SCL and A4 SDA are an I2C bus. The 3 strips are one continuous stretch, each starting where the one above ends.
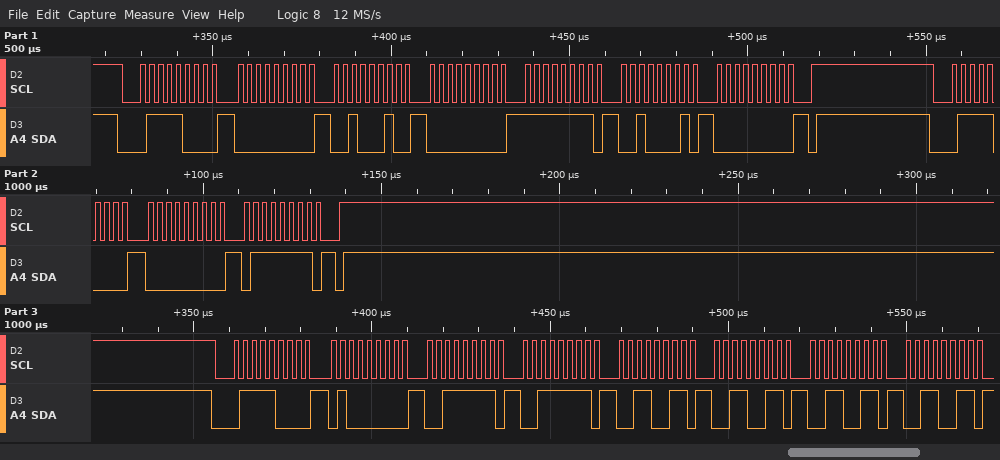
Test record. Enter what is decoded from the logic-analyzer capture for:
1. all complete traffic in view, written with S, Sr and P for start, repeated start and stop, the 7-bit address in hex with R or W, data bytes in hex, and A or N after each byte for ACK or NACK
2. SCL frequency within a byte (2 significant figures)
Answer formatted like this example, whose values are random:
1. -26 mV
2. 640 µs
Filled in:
1. S 3CW A 00 A 22 A 00 A FF A 21 A 00 A P S 3CW A 00 A 7F A P S 3CW A 40 A 3F A 3F A 33 A 33 A 33 A 33 A
2. 400 kHz
